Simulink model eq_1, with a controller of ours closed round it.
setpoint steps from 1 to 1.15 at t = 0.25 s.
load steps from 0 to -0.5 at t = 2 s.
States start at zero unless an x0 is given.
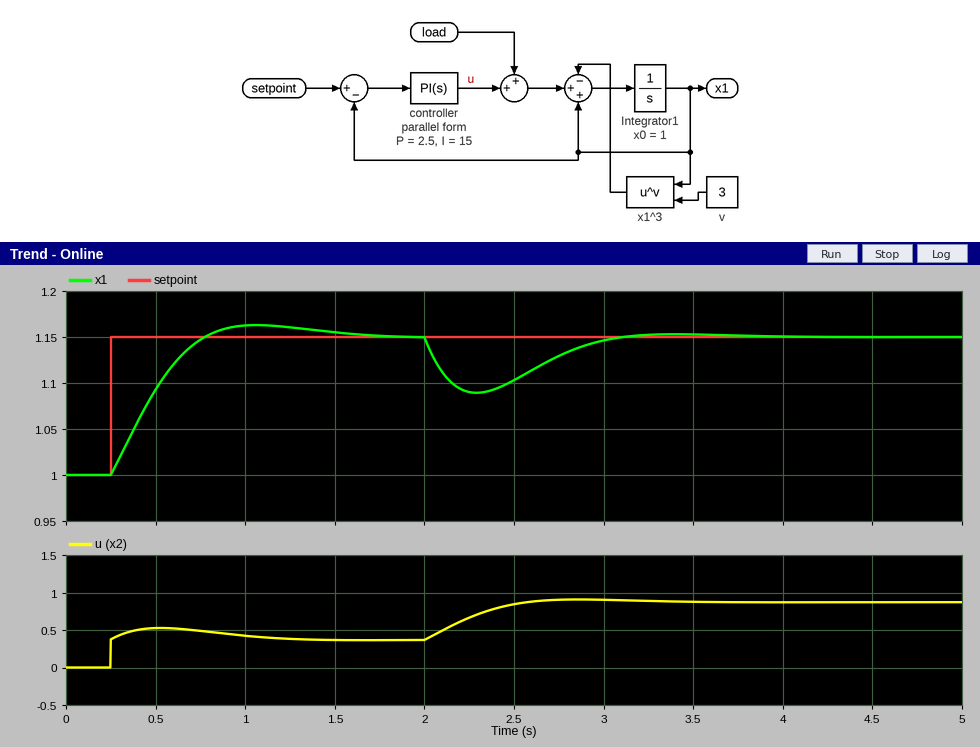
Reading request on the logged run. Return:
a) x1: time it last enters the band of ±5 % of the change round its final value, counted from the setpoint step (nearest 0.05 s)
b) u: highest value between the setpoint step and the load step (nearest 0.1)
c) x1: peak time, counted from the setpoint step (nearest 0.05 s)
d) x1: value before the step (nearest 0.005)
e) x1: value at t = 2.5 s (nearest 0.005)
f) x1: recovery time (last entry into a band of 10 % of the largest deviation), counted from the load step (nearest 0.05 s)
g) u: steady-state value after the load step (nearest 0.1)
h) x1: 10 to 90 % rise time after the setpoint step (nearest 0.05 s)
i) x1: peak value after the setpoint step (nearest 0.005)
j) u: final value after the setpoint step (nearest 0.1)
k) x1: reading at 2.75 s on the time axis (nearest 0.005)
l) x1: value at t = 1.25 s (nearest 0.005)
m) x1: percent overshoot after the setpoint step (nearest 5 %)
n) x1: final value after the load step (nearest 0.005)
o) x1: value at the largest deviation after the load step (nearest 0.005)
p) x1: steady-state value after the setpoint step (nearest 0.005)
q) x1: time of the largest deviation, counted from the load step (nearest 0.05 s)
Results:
1.15 s
0.5
0.80 s
1.000
1.105
0.95 s
0.9
0.40 s
1.165
0.4
1.130
1.160
10 %
1.150
1.090
1.150
0.30 s
